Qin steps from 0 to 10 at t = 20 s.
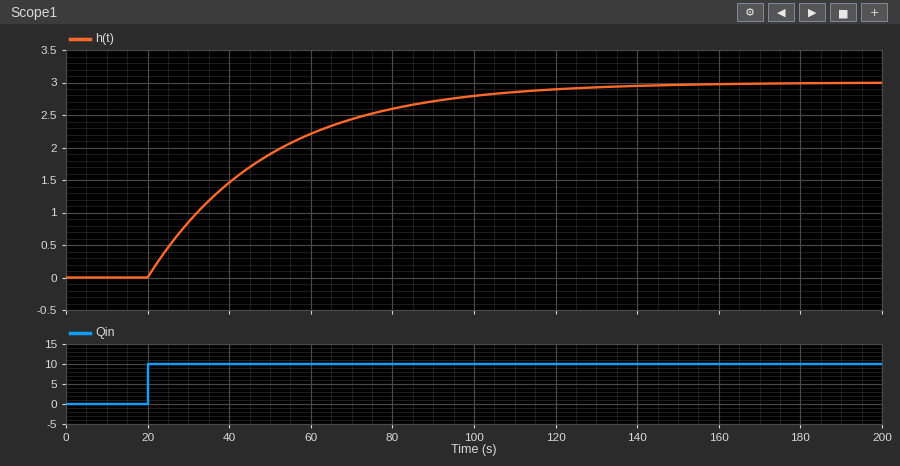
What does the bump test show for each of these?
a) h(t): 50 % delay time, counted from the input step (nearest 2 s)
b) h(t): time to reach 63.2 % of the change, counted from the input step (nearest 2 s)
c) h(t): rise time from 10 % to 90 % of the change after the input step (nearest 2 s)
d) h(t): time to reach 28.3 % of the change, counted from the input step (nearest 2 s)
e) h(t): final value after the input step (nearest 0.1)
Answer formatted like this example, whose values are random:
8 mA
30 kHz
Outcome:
20 s
30 s
66 s
10 s
3.0
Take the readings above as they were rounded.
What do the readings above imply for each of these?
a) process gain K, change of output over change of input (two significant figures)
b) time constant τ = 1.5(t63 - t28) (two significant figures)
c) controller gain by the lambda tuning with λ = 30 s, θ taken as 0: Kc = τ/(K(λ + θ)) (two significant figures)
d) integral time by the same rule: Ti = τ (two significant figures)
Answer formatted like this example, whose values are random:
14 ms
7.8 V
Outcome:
0.30
30 s
3.3
30 s
